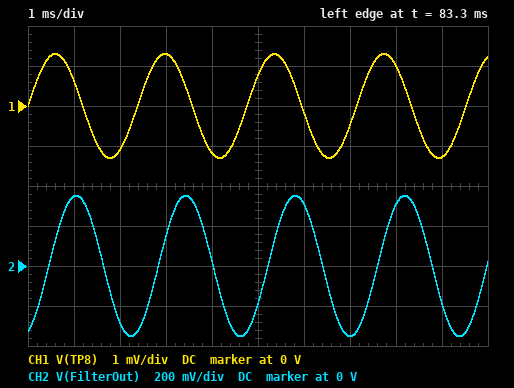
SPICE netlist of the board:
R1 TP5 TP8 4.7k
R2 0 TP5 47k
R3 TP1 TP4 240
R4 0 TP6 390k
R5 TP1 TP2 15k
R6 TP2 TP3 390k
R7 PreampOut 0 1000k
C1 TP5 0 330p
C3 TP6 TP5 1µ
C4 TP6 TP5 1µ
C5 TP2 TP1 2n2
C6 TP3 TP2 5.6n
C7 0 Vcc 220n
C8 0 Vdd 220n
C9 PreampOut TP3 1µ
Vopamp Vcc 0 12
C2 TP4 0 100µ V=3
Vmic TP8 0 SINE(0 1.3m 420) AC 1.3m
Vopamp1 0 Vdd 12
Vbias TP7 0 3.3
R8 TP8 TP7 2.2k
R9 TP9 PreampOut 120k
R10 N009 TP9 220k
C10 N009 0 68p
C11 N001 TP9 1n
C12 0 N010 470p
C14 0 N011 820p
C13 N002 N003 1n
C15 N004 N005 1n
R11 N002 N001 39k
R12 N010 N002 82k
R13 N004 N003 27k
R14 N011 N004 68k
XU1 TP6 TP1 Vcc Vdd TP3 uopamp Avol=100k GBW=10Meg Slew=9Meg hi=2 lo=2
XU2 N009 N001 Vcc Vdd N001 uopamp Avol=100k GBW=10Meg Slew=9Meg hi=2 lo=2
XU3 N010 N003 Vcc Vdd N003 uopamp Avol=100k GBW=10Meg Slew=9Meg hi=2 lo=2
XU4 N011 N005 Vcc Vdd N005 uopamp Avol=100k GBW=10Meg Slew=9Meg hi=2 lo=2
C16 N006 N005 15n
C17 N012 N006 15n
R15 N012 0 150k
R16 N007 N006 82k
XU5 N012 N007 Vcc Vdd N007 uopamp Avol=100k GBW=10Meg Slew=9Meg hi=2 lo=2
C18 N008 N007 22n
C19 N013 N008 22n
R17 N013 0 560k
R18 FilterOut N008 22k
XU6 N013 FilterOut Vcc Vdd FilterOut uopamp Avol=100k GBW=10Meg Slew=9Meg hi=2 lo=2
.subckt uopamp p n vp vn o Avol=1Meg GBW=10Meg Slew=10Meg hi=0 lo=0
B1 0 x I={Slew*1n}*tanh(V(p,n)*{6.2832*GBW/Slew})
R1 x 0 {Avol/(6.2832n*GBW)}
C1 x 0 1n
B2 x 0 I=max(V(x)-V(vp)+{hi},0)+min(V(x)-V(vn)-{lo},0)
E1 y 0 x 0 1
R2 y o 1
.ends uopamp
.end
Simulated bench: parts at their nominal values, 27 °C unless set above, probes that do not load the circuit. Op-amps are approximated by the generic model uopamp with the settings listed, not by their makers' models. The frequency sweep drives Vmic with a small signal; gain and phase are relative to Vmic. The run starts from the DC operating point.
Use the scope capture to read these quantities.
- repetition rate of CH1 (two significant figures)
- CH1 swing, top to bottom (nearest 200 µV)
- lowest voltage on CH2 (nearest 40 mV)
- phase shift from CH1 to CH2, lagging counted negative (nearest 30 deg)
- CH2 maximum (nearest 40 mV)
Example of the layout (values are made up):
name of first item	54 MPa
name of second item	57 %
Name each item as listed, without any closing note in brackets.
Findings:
repetition rate of CH1	420 Hz
CH1 swing, top to bottom	2.6 mV
lowest voltage on CH2	-360 mV
phase shift from CH1 to CH2, lagging counted negative	-60 deg
CH2 maximum	360 mV
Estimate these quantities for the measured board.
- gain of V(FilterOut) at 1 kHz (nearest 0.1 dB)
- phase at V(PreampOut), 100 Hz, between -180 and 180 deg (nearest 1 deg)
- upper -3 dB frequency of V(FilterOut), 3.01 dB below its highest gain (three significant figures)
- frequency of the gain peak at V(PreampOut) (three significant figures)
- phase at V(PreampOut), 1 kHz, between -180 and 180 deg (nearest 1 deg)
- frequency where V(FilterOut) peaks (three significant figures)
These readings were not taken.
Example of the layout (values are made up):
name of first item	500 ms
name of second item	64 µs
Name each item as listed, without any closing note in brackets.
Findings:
gain of V(FilterOut) at 1 kHz	42.3 dB
phase at V(PreampOut), 100 Hz, between -180 and 180 deg	-47 deg
upper -3 dB frequency of V(FilterOut), 3.01 dB below its highest gain	115 Hz
frequency of the gain peak at V(PreampOut)	21.9 Hz
phase at V(PreampOut), 1 kHz, between -180 and 180 deg	-62 deg
frequency where V(FilterOut) peaks	71.8 Hz
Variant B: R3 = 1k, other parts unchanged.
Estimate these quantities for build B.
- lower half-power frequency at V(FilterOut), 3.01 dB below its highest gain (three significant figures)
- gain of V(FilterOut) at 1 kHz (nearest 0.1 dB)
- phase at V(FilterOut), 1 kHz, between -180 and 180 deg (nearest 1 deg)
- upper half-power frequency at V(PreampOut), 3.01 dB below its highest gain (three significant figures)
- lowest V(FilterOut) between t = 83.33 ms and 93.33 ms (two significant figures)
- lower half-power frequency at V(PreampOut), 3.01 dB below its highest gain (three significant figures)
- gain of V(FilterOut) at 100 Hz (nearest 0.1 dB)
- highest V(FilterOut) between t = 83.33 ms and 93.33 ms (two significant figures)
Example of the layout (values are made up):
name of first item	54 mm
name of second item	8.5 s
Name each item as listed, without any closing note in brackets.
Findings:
lower half-power frequency at V(FilterOut), 3.01 dB below its highest gain	60.2 Hz
gain of V(FilterOut) at 1 kHz	30.1 dB
phase at V(FilterOut), 1 kHz, between -180 and 180 deg	-109 deg
upper half-power frequency at V(PreampOut), 3.01 dB below its highest gain	76.3 Hz
lowest V(FilterOut) between t = 83.33 ms and 93.33 ms	-86 mV
lower half-power frequency at V(PreampOut), 3.01 dB below its highest gain	1.56 Hz
gain of V(FilterOut) at 100 Hz	47.6 dB
highest V(FilterOut) between t = 83.33 ms and 93.33 ms	86 mV
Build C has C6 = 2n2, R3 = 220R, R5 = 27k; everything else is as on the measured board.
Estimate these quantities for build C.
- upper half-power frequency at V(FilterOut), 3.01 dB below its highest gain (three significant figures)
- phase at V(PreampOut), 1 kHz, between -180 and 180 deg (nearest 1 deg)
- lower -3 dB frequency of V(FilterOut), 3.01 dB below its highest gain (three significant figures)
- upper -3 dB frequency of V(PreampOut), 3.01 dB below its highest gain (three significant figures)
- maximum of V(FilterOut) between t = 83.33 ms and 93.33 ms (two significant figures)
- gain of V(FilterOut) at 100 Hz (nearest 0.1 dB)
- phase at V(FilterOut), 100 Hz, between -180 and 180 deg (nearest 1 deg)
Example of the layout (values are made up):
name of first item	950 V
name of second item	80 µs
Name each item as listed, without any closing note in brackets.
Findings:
upper half-power frequency at V(FilterOut), 3.01 dB below its highest gain	175 Hz
phase at V(PreampOut), 1 kHz, between -180 and 180 deg	-66 deg
lower -3 dB frequency of V(FilterOut), 3.01 dB below its highest gain	61.1 Hz
upper -3 dB frequency of V(PreampOut), 3.01 dB below its highest gain	199 Hz
maximum of V(FilterOut) between t = 83.33 ms and 93.33 ms	910 mV
gain of V(FilterOut) at 100 Hz	64.3 dB
phase at V(FilterOut), 100 Hz, between -180 and 180 deg	82 deg
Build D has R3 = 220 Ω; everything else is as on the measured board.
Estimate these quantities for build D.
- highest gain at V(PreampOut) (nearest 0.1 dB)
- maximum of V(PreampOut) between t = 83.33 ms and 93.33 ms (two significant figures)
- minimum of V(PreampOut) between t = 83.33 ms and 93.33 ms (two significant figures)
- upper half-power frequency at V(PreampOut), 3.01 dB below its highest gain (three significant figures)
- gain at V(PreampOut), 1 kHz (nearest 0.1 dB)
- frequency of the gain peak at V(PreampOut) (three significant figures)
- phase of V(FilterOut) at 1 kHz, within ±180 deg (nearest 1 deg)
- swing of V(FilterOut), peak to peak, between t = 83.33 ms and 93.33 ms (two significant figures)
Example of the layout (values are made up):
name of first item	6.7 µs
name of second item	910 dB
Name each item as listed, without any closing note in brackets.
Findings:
highest gain at V(PreampOut)	63.4 dB
maximum of V(PreampOut) between t = 83.33 ms and 93.33 ms	380 mV
minimum of V(PreampOut) between t = 83.33 ms and 93.33 ms	-380 mV
upper half-power frequency at V(PreampOut), 3.01 dB below its highest gain	86.6 Hz
gain at V(PreampOut), 1 kHz	43.1 dB
frequency of the gain peak at V(PreampOut)	22.8 Hz
phase of V(FilterOut) at 1 kHz, within ±180 deg	-110 deg
swing of V(FilterOut), peak to peak, between t = 83.33 ms and 93.33 ms	770 mV
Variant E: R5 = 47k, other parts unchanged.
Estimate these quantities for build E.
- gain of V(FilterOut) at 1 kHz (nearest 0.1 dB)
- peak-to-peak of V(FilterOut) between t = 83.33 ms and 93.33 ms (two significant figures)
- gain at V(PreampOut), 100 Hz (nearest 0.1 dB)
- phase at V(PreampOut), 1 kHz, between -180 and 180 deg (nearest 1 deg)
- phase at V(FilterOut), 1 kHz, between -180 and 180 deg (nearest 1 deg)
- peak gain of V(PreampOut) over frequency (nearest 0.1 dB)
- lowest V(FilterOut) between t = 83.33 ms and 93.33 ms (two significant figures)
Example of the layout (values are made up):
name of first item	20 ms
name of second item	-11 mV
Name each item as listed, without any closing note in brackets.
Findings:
gain of V(FilterOut) at 1 kHz	47.0 dB
peak-to-peak of V(FilterOut) between t = 83.33 ms and 93.33 ms	930 mV
gain at V(PreampOut), 100 Hz	59.7 dB
phase at V(PreampOut), 1 kHz, between -180 and 180 deg	-55 deg
phase at V(FilterOut), 1 kHz, between -180 and 180 deg	-103 deg
peak gain of V(PreampOut) over frequency	63.4 dB
lowest V(FilterOut) between t = 83.33 ms and 93.33 ms	-460 mV
